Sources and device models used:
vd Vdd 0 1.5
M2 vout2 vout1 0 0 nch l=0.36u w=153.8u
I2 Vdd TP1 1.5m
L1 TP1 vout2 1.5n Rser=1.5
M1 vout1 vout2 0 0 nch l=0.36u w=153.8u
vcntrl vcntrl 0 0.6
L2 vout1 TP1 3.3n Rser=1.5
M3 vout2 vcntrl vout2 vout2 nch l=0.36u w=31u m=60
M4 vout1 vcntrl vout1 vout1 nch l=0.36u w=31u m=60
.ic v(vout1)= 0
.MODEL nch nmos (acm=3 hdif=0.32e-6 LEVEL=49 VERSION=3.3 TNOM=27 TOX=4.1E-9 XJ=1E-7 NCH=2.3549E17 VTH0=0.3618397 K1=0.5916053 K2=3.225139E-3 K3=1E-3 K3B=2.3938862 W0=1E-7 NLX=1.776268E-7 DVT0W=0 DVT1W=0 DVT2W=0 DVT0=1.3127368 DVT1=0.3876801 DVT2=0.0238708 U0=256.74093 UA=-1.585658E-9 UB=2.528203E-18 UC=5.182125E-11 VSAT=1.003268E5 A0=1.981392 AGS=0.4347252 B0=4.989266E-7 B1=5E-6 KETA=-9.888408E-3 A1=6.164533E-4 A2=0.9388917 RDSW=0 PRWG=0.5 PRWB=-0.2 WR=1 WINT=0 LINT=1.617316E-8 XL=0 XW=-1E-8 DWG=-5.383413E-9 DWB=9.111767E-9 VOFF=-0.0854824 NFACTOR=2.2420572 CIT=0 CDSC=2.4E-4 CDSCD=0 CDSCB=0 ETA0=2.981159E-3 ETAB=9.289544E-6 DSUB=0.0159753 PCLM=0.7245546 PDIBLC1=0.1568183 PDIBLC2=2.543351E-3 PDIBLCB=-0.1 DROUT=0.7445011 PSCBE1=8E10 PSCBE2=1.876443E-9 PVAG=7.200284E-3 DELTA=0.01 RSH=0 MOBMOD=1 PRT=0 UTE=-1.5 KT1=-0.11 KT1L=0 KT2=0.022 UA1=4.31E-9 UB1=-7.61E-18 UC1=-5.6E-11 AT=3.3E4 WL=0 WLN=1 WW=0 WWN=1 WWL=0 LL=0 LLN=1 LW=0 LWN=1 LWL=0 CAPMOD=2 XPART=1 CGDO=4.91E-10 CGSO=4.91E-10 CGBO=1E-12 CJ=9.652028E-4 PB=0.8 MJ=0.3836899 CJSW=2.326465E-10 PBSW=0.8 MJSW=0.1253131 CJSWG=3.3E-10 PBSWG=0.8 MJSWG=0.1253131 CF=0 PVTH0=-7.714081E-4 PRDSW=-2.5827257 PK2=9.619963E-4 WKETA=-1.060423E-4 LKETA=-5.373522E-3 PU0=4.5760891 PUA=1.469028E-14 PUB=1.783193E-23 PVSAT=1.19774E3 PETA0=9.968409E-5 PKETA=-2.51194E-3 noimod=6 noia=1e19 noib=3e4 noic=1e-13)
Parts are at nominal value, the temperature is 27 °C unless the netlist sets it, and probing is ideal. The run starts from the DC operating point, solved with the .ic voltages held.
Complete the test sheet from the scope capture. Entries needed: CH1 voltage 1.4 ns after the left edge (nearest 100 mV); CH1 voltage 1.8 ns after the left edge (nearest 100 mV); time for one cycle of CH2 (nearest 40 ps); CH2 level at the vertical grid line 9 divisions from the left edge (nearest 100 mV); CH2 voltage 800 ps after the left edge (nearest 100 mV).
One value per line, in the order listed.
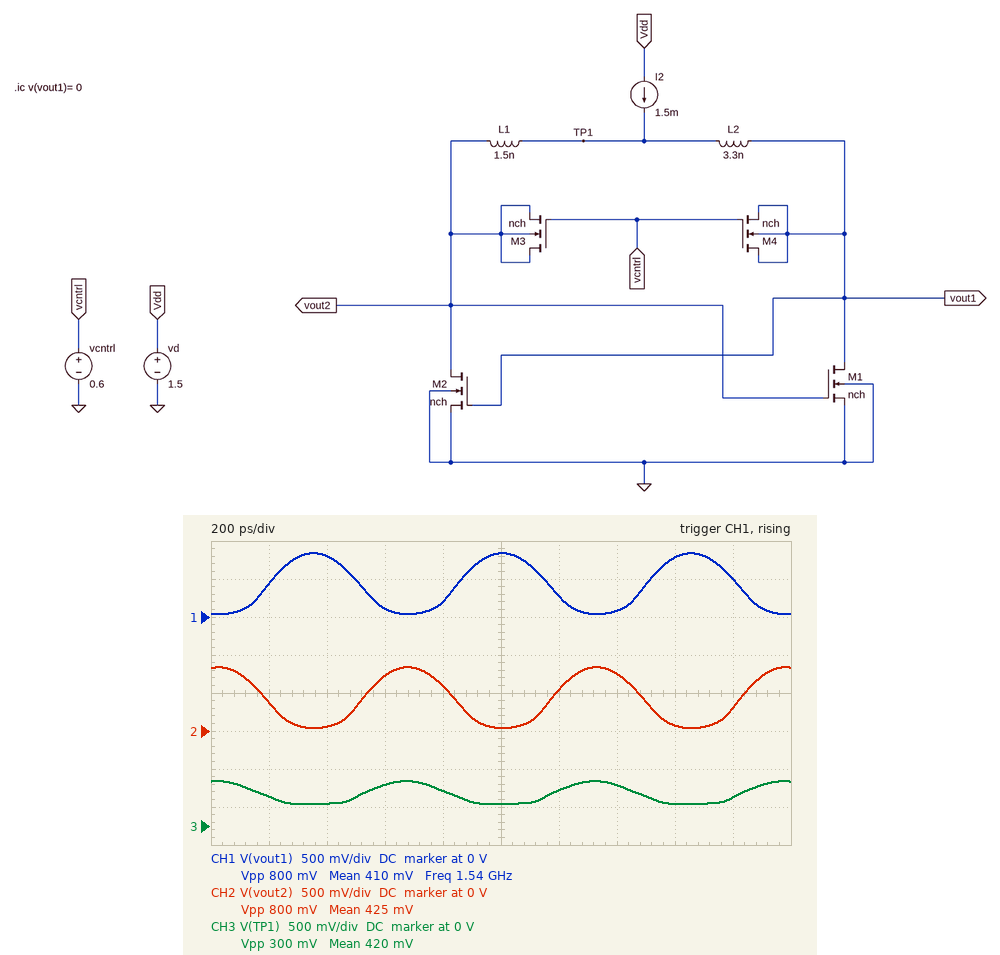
100 mV
500 mV
640 ps
300 mV
600 mV
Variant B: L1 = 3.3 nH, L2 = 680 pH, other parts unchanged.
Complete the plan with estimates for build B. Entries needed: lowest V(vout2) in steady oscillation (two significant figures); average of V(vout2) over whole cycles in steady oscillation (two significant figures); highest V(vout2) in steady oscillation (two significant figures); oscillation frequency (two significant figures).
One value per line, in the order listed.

67 mV
410 mV
780 mV
1.7 GHz
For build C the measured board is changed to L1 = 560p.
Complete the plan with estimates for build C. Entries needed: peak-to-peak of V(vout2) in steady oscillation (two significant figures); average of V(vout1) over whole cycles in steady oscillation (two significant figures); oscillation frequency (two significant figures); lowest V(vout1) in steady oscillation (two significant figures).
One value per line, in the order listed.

700 mV
410 mV
1.7 GHz
73 mV
